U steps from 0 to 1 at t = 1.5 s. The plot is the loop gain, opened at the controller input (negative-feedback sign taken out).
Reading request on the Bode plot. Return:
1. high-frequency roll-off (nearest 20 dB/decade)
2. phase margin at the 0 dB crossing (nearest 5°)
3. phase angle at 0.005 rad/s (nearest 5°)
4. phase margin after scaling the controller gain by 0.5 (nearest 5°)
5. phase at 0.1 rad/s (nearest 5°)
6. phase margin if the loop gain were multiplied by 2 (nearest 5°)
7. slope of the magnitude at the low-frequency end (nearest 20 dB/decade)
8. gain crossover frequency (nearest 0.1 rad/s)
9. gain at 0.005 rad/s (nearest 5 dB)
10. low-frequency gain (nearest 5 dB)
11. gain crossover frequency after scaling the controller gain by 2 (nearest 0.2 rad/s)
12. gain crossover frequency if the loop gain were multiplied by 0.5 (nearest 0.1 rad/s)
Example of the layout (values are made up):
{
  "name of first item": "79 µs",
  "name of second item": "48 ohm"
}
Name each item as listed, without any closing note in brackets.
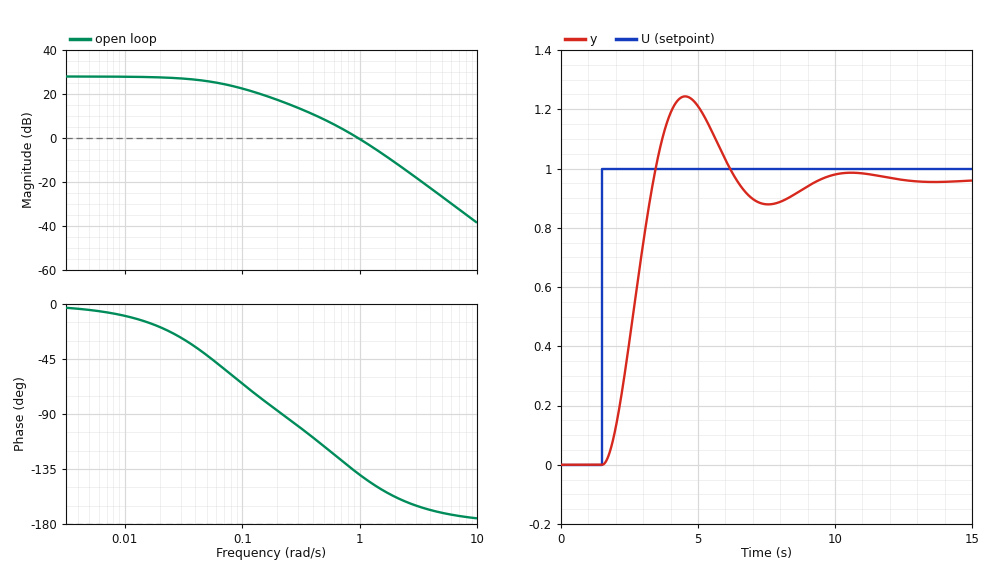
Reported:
{
  "high-frequency roll-off": "-40 dB/decade",
  "phase margin at the 0 dB crossing": "40°",
  "phase angle at 0.005 rad/s": "-5°",
  "phase margin after scaling the controller gain by 0.5": "55°",
  "phase at 0.1 rad/s": "-65°",
  "phase margin if the loop gain were multiplied by 2": "30°",
  "slope of the magnitude at the low-frequency end": "0 dB/decade",
  "gain crossover frequency": "1.0 rad/s",
  "gain at 0.005 rad/s": "30 dB",
  "low-frequency gain": "30 dB",
  "gain crossover frequency after scaling the controller gain by 2": "1.4 rad/s",
  "gain crossover frequency if the loop gain were multiplied by 0.5": "0.6 rad/s"
}
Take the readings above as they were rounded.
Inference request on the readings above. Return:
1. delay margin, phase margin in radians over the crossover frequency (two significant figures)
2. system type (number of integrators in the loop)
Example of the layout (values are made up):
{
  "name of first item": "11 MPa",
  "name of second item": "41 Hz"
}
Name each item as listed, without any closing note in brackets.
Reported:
{
  "delay margin, phase margin in radians over the crossover frequency": "0.70 s",
  "system type": "0"
}
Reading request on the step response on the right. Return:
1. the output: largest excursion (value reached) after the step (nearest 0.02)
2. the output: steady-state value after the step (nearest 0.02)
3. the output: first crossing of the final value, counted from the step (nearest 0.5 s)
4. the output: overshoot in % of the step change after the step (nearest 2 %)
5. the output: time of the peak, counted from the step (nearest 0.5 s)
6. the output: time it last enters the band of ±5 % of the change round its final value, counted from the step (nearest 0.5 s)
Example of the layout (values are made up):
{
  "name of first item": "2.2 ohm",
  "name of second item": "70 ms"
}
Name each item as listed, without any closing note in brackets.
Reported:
{
  "the output: largest excursion (value reached) after the step": "1.24",
  "the output: steady-state value after the step": "0.96",
  "the output: first crossing of the final value, counted from the step": "2.0 s",
  "the output: overshoot in % of the step change after the step": "30 %",
  "the output: time of the peak, counted from the step": "3.0 s",
  "the output: time it last enters the band of ±5 % of the change round its final value, counted from the step": "7.0 s"
}
